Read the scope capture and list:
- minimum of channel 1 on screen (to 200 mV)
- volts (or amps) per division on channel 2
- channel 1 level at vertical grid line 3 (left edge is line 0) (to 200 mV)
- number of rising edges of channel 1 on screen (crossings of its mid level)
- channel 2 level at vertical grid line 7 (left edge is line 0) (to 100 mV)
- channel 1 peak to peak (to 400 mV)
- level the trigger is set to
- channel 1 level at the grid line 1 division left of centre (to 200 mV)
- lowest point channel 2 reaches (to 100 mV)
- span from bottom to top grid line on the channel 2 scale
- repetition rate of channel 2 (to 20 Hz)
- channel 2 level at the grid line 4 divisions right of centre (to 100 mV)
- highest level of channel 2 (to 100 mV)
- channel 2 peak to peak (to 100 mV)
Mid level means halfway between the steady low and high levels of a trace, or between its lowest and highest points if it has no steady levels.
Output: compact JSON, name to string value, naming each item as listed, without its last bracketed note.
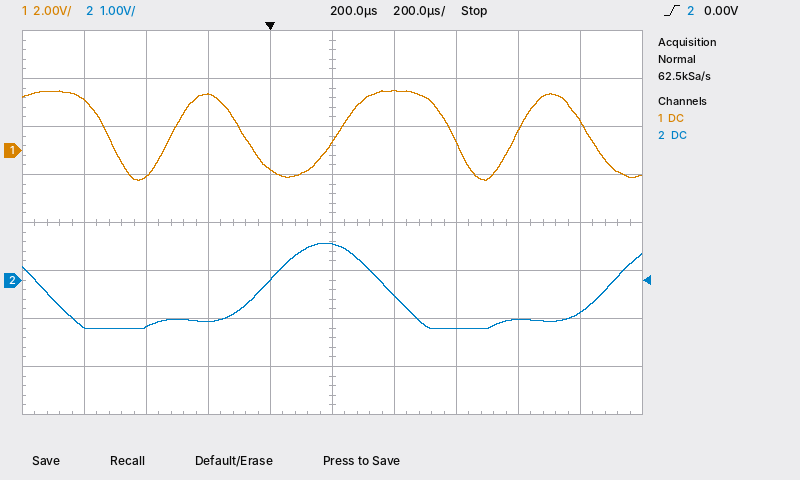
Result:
{"minimum of channel 1 on screen": "-1.2 V", "volts (or amps) per division on channel 2": "1 V", "channel 1 level at vertical grid line 3 (left edge is line 0)": "2.4 V", "number of rising edges of channel 1 on screen": "3", "channel 2 level at vertical grid line 7 (left edge is line 0)": "-1.0 V", "channel 1 peak to peak": "3.6 V", "level the trigger is set to": "0.00 V", "channel 1 level at the grid line 1 division left of centre": "-800 mV", "lowest point channel 2 reaches": "-1.0 V", "span from bottom to top grid line on the channel 2 scale": "8 V", "repetition rate of channel 2": "900 Hz", "channel 2 level at the grid line 4 divisions right of centre": "-700 mV", "highest level of channel 2": "800 mV", "channel 2 peak to peak": "1.8 V"}
